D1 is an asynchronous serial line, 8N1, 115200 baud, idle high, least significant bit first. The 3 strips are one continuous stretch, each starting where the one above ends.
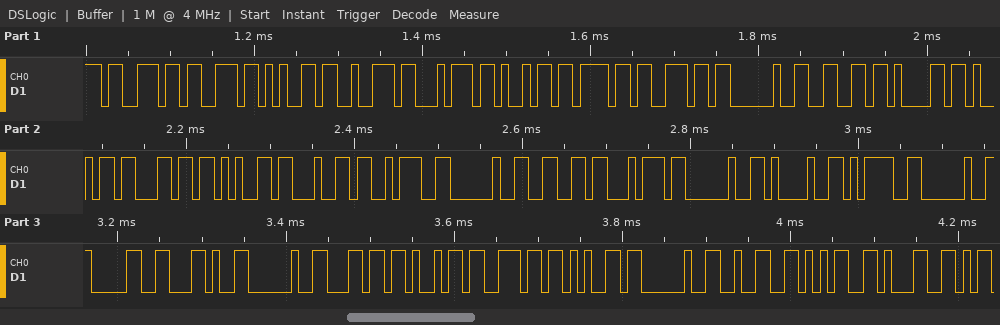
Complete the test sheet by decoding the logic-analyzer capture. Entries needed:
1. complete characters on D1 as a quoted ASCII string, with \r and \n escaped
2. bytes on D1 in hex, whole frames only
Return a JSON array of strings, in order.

["\"ssertion failed: ft != 0, line 251\"", "73 73 65 72 74 69 6F 6E 20 66 61 69 6C 65 64 3A 20 66 74 20 21 3D 20 30 2C 20 6C 69 6E 65 20 32 35 31"]
